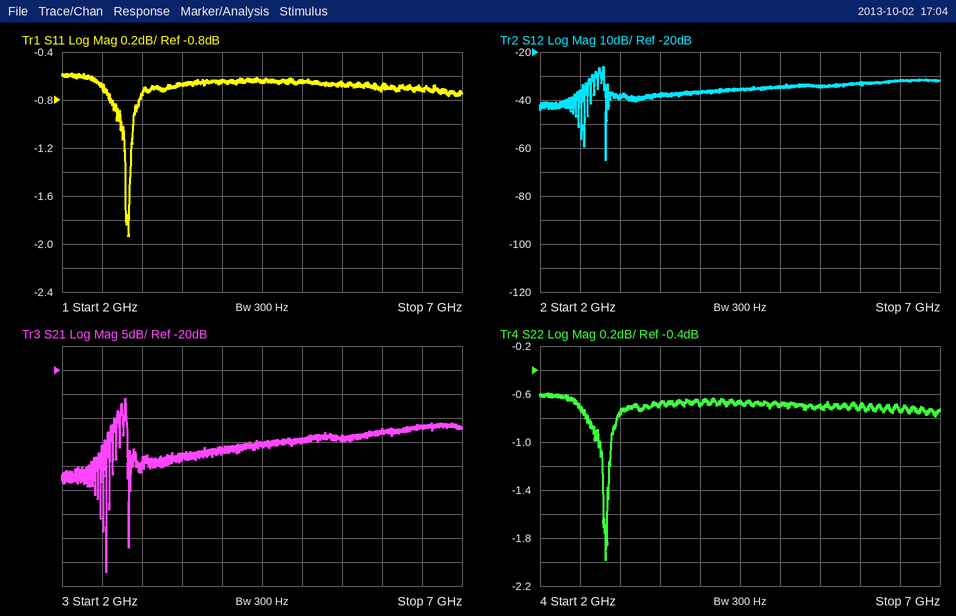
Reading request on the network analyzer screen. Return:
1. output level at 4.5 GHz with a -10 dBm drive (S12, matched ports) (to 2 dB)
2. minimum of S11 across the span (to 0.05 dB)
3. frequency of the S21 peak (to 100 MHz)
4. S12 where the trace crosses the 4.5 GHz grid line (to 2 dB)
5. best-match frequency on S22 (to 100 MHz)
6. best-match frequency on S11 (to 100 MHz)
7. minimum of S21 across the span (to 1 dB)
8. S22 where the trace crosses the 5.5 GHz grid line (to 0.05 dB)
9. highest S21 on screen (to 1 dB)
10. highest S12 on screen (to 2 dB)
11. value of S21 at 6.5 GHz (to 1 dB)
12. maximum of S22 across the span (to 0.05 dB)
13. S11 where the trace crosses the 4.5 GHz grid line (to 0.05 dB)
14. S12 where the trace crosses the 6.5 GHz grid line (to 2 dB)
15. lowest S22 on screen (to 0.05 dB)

-46 dBm
-1.95 dB
2.8 GHz
-36 dB
2.8 GHz
2.8 GHz
-62 dB
-0.70 dB
-26 dB
-26 dB
-32 dB
-0.60 dB
-0.65 dB
-32 dB
-2.00 dB
